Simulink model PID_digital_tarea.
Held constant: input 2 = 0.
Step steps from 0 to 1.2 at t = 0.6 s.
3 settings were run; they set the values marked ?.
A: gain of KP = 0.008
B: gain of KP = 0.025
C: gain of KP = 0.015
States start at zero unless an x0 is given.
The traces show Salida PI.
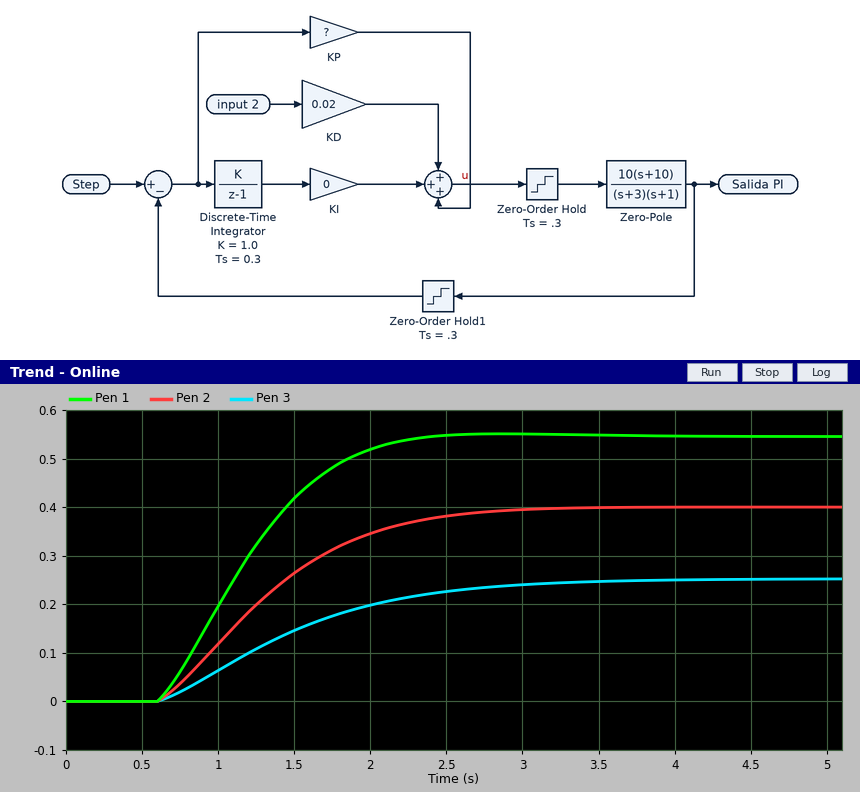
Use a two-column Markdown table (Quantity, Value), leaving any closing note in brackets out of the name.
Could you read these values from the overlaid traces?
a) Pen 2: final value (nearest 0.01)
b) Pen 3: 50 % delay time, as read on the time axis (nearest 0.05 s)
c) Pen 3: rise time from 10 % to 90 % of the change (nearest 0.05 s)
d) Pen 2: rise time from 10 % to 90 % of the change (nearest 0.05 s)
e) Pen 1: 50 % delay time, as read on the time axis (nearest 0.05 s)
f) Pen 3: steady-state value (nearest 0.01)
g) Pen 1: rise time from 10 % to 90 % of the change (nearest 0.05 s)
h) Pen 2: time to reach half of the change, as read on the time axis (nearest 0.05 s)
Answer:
| Quantity | Value |
|---|---|
| Pen 2: final value | 0.40 |
| Pen 3: 50 % delay time, as read on the time axis | 1.35 s |
| Pen 3: rise time from 10 % to 90 % of the change | 1.75 s |
| Pen 2: rise time from 10 % to 90 % of the change | 1.40 s |
| Pen 1: 50 % delay time, as read on the time axis | 1.15 s |
| Pen 3: steady-state value | 0.25 |
| Pen 1: rise time from 10 % to 90 % of the change | 1.05 s |
| Pen 2: time to reach half of the change, as read on the time axis | 1.25 s |
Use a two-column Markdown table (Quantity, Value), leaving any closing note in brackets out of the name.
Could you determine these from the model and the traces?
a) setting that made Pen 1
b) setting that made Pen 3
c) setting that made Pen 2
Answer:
| Quantity | Value |
|---|---|
| setting that made Pen 1 | B |
| setting that made Pen 3 | A |
| setting that made Pen 2 | C |
